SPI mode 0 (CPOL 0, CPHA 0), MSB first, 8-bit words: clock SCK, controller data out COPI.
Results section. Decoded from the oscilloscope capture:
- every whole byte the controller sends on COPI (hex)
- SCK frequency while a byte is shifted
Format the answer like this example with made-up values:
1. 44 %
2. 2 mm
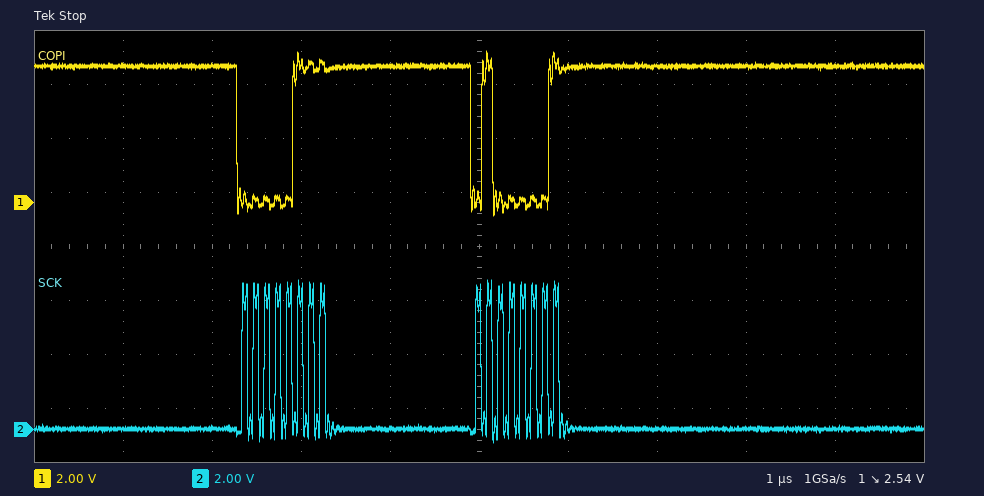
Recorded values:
1. 0x07 0x41
2. 8 MHz
